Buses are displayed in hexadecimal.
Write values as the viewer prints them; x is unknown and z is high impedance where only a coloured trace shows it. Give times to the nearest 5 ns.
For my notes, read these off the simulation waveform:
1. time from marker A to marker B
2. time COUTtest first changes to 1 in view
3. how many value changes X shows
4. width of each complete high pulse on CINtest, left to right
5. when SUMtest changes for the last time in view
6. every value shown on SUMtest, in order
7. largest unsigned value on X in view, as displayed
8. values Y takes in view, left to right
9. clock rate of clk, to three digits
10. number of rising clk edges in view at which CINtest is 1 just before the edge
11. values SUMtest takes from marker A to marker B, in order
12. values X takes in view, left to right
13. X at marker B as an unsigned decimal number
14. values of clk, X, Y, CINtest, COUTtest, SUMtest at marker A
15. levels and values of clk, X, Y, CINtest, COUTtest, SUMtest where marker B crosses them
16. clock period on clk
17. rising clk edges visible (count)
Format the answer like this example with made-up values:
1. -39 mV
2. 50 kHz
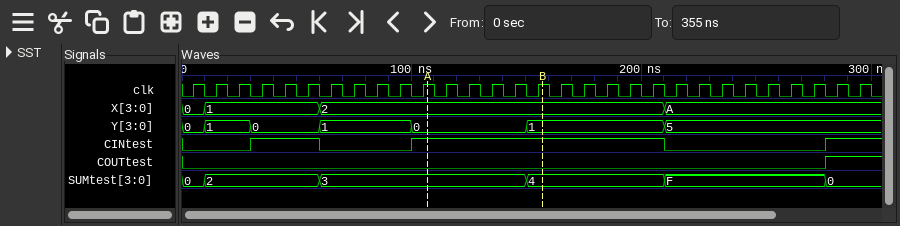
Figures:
1. 50 ns
2. 280 ns
3. 3
4. 30 ns, 110 ns
5. 280 ns
6. 0, 2, 3, 4, F, 0
7. A
8. 0, 1, 0, 1, 0, 1, 5
9. 100 MHz
10. 16
11. 3, 4
12. 0, 1, 2, A
13. 2
14. clk=1, X=2, Y=0, CINtest=1, COUTtest=0, SUMtest=3
15. clk=1, X=2, Y=1, CINtest=1, COUTtest=0, SUMtest=4
16. 10 ns
17. 30
